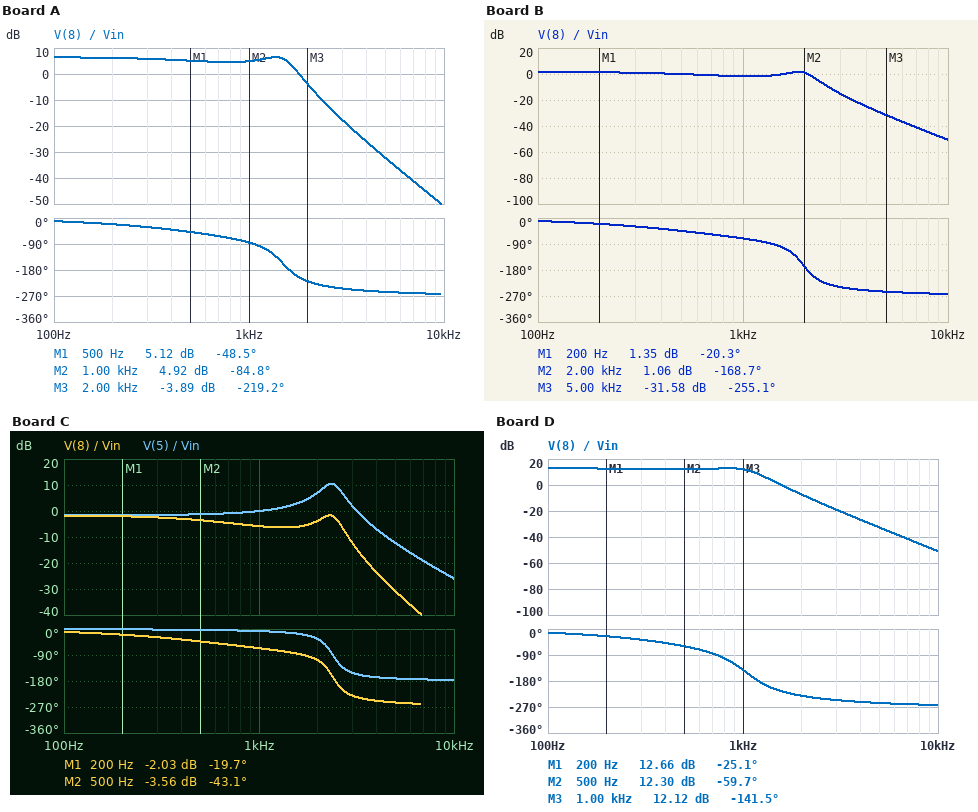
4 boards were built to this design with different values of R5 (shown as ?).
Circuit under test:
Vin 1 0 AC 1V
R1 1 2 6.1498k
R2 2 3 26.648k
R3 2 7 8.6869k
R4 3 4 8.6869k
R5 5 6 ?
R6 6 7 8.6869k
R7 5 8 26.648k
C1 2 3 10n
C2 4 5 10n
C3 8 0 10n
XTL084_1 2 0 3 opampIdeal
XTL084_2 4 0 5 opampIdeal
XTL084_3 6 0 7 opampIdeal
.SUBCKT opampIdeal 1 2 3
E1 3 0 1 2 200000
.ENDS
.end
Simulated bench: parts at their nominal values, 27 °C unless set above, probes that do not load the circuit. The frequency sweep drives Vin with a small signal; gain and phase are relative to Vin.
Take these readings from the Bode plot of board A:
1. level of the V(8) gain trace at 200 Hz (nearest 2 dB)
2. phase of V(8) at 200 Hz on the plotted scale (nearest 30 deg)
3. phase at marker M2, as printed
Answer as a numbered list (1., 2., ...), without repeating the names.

1. 6 dB
2. -30 deg
3. -84.8 deg
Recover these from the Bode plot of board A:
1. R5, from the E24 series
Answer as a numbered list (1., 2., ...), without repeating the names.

1. 13 kΩ
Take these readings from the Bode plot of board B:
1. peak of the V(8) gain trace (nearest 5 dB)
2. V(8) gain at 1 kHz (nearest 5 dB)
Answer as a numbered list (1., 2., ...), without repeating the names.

1. 0 dB
2. 0 dB
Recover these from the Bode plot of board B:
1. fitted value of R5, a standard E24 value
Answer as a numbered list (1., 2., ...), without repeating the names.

1. 7.5 kΩ
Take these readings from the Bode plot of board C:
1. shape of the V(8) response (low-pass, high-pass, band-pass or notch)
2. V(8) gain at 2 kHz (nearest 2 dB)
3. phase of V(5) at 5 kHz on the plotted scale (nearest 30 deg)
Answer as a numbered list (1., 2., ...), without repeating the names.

1. low-pass
2. -4 dB
3. -180 deg
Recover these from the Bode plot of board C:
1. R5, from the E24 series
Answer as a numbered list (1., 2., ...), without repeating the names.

1. 5.1 kΩ
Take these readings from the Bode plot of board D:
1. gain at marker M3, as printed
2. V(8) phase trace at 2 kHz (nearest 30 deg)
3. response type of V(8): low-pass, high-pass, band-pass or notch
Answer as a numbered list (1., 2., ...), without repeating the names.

1. 12.12 dB
2. -240 deg
3. low-pass
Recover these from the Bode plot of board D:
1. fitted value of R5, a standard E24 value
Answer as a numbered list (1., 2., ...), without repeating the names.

1. 27 kΩ
